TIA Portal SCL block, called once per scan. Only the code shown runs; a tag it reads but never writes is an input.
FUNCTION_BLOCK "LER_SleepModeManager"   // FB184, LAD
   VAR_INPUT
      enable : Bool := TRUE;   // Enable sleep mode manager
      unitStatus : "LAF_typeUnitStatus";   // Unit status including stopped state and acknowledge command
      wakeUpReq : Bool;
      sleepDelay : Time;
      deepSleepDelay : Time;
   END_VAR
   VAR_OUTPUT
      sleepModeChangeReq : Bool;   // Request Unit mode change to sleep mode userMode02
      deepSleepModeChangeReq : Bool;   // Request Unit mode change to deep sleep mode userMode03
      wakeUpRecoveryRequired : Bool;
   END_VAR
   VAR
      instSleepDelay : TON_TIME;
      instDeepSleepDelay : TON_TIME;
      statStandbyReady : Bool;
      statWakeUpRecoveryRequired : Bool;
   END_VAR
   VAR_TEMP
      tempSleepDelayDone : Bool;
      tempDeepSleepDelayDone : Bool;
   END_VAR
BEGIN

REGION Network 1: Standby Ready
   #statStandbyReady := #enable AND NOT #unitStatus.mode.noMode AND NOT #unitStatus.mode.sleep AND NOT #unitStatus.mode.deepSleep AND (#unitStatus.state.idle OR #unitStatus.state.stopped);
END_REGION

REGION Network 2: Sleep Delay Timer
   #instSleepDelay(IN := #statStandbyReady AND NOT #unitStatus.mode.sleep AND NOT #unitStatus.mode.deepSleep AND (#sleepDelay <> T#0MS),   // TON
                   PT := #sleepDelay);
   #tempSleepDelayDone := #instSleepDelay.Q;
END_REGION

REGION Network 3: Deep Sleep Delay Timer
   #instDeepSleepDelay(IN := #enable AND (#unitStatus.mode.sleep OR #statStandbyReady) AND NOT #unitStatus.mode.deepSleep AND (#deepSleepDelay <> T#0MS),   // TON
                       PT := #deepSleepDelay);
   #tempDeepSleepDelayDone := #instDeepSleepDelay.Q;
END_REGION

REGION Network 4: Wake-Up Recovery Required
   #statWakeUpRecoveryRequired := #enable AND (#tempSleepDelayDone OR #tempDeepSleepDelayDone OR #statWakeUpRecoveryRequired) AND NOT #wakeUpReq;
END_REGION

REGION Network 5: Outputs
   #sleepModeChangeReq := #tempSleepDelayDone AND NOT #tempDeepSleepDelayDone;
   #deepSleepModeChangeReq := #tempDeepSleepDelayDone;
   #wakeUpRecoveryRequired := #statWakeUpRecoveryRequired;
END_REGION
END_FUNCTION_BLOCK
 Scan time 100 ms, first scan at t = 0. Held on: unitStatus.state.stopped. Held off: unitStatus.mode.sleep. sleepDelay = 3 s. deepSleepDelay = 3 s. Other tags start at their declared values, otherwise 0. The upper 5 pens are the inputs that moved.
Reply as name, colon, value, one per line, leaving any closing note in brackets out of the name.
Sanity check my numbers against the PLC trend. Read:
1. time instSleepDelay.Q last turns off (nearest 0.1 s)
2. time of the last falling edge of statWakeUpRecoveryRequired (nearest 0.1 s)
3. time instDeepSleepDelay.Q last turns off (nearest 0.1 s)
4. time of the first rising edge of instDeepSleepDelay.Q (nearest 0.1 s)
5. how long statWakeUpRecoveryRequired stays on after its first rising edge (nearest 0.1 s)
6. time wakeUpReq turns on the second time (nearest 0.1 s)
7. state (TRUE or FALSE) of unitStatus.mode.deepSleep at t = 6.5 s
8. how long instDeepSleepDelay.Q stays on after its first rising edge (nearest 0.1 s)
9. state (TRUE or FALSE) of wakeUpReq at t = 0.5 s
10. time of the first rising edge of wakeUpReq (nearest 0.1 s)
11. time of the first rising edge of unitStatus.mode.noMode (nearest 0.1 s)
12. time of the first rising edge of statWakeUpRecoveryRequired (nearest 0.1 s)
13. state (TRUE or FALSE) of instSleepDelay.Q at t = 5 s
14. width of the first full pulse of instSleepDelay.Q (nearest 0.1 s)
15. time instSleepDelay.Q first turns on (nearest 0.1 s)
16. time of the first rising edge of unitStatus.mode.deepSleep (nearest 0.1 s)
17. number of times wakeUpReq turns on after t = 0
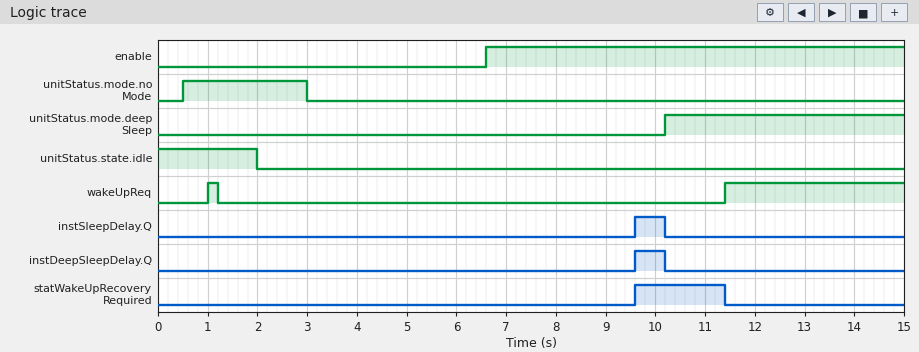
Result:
time instSleepDelay.Q last turns off: 10.2 s
time of the last falling edge of statWakeUpRecoveryRequired: 11.4 s
time instDeepSleepDelay.Q last turns off: 10.2 s
time of the first rising edge of instDeepSleepDelay.Q: 9.6 s
how long statWakeUpRecoveryRequired stays on after its first rising edge: 1.8 s
time wakeUpReq turns on the second time: 11.4 s
state (TRUE or FALSE) of unitStatus.mode.deepSleep at t = 6.5 s: FALSE
how long instDeepSleepDelay.Q stays on after its first rising edge: 0.6 s
state (TRUE or FALSE) of wakeUpReq at t = 0.5 s: FALSE
time of the first rising edge of wakeUpReq: 1.0 s
time of the first rising edge of unitStatus.mode.noMode: 0.5 s
time of the first rising edge of statWakeUpRecoveryRequired: 9.6 s
state (TRUE or FALSE) of instSleepDelay.Q at t = 5 s: FALSE
width of the first full pulse of instSleepDelay.Q: 0.6 s
time instSleepDelay.Q first turns on: 9.6 s
time of the first rising edge of unitStatus.mode.deepSleep: 10.2 s
number of times wakeUpReq turns on after t = 0: 2
